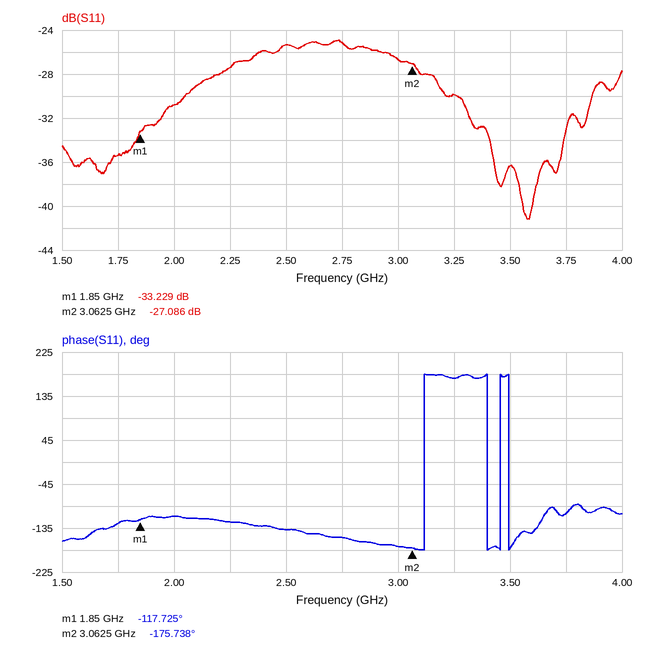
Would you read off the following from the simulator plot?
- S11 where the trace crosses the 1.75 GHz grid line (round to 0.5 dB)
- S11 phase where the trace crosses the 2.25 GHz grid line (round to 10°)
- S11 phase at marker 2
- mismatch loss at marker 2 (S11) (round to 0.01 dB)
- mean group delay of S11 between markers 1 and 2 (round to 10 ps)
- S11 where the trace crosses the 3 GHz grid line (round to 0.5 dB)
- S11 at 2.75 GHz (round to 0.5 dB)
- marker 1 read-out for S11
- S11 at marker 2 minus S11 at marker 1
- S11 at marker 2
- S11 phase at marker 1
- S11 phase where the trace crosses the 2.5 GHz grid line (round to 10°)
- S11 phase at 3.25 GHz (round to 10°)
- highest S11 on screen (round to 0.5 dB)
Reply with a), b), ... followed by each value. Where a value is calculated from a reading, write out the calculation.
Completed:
a) -35.5 dB
b) -120°
c) -175.738°
d) −10 log10(1 − 10^(-27.086/10)) ≈ 0.01 dB
e) −(-175.738° − (-117.725°))/(360° × 1.2125 GHz) ≈ 133 ps, so 130 ps to the nearest 10 ps
f) -26.5 dB
g) -25.0 dB
h) -33.229 dB
i) -27.086 − (-33.229) = 6.143 dB
j) -27.086 dB
k) -117.725°
l) -140°
m) 170°
n) -25.0 dB
